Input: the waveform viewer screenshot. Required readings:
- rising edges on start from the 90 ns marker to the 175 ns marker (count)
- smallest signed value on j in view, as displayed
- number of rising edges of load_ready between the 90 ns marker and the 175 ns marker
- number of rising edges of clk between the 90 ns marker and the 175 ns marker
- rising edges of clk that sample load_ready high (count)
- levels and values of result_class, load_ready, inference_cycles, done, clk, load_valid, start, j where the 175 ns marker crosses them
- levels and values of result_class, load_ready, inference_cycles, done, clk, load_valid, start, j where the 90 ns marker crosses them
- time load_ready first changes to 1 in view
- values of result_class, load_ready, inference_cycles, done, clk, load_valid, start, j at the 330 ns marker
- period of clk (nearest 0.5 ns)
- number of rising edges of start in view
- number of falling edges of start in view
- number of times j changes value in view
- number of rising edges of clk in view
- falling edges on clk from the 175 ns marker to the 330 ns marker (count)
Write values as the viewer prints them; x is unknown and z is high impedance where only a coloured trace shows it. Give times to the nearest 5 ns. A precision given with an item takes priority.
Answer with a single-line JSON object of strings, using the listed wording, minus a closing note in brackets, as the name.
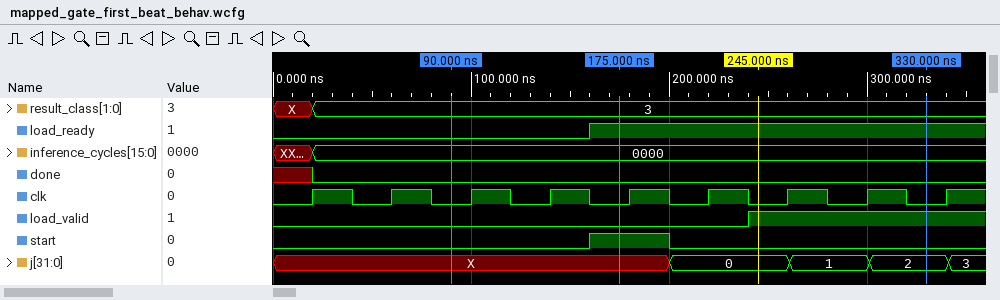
{"rising edges on start from the 90 ns marker to the 175 ns marker": "1", "smallest signed value on j in view, as displayed": "0", "number of rising edges of load_ready between the 90 ns marker and the 175 ns marker": "1", "number of rising edges of clk between the 90 ns marker and the 175 ns marker": "2", "rising edges of clk that sample load_ready high": "5", "levels and values of result_class, load_ready, inference_cycles, done, clk, load_valid, start, j where the 175 ns marker crosses them": "result_class=3, load_ready=1, inference_cycles=0000, done=0, clk=0, load_valid=0, start=1, j=X", "levels and values of result_class, load_ready, inference_cycles, done, clk, load_valid, start, j where the 90 ns marker crosses them": "result_class=3, load_ready=0, inference_cycles=0000, done=0, clk=0, load_valid=0, start=0, j=X", "time load_ready first changes to 1 in view": "160 ns", "values of result_class, load_ready, inference_cycles, done, clk, load_valid, start, j at the 330 ns marker": "result_class=3, load_ready=1, inference_cycles=0000, done=0, clk=0, load_valid=1, start=0, j=2", "period of clk": "40 ns", "number of rising edges of start in view": "1", "number of falling edges of start in view": "1", "number of times j changes value in view": "4", "number of rising edges of clk in view": "9", "falling edges on clk from the 175 ns marker to the 330 ns marker": "4"}
